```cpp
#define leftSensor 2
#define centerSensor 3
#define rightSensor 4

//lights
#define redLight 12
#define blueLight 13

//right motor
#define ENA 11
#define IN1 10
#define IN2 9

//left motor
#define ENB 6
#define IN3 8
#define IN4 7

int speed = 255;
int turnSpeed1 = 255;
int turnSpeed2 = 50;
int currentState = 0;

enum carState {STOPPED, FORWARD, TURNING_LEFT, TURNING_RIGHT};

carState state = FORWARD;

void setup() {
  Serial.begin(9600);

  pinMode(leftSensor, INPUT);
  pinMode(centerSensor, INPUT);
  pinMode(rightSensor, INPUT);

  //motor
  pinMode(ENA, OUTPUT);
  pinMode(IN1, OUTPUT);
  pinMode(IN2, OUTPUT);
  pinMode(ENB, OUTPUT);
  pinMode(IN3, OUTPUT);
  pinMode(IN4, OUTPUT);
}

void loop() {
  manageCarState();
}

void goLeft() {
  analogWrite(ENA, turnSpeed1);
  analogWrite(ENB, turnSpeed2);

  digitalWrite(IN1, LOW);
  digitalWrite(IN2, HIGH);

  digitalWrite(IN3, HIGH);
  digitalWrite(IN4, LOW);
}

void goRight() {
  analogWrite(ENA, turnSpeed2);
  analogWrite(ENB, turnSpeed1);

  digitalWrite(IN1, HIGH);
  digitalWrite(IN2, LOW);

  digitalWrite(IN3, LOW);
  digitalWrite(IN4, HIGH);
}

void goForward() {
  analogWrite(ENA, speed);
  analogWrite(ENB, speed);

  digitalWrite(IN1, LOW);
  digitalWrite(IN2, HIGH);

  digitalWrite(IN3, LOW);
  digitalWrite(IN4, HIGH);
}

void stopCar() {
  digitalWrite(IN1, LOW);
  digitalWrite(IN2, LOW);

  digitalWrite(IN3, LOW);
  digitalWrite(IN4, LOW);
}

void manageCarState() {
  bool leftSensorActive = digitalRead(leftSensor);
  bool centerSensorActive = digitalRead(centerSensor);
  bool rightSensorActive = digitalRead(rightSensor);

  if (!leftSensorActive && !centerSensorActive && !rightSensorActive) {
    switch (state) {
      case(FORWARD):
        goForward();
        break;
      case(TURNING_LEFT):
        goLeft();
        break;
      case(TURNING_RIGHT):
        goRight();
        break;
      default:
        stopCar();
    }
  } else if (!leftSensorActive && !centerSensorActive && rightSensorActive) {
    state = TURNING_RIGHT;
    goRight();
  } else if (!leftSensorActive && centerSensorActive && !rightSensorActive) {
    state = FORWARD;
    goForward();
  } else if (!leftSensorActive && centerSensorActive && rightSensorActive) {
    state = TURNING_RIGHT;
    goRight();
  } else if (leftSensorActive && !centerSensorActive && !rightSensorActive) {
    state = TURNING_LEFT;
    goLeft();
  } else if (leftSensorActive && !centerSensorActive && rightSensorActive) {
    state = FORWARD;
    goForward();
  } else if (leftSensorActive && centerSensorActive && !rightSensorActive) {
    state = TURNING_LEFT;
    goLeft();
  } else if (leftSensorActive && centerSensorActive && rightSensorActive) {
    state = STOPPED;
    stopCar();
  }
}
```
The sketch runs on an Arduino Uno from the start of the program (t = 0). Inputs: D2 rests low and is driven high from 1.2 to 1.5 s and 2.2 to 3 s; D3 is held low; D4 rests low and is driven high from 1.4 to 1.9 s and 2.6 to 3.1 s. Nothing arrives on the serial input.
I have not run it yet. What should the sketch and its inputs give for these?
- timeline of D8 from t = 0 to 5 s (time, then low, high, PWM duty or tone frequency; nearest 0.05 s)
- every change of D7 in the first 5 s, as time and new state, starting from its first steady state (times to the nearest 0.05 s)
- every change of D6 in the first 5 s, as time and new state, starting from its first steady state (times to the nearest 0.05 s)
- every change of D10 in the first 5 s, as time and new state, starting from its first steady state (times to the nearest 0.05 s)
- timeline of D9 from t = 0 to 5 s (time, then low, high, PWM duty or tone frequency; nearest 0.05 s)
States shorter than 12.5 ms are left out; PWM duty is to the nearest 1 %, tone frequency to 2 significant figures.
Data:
0 s low; 1.2 s high; 1.4 s low; 2.2 s high; 2.6 s low
0 s high; 1.2 s low; 1.4 s high; 2.2 s low; 2.6 s high
0 s high; 1.2 s PWM 20 %; 1.4 s high; 2.2 s PWM 20 %; 2.6 s high
0 s low; 1.5 s high; 2.2 s low; 3 s high
0 s high; 1.5 s low; 2.2 s high; 3 s low
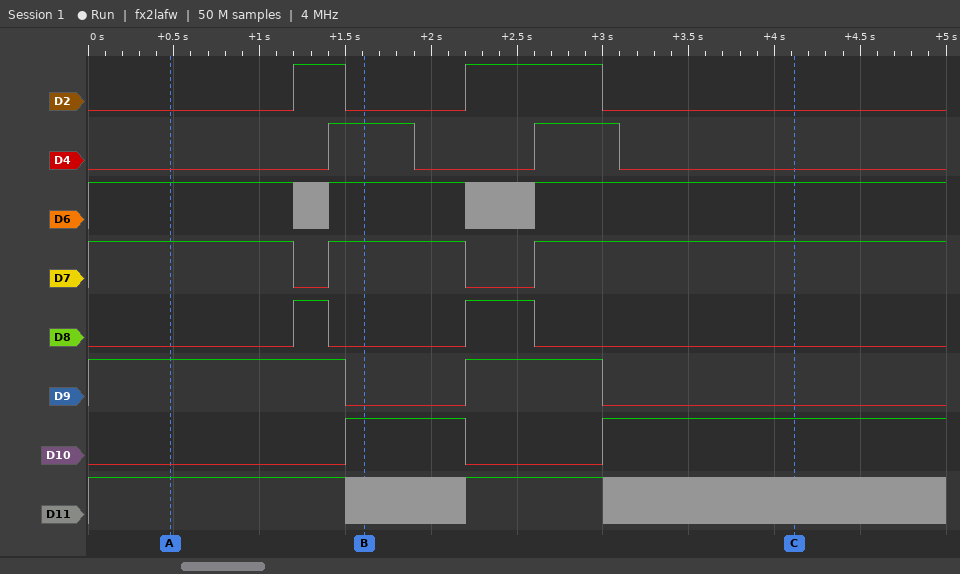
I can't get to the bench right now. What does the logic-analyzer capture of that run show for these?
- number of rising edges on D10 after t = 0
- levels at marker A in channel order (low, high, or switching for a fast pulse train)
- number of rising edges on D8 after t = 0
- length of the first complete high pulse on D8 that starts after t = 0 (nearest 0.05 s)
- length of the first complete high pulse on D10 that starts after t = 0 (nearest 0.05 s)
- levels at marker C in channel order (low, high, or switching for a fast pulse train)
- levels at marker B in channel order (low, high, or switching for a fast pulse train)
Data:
2
D2 low, D4 low, D6 high, D7 high, D8 low, D9 high, D10 low, D11 high
2
0.20 s
0.70 s
D2 low, D4 low, D6 high, D7 high, D8 low, D9 low, D10 high, D11 switching
D2 low, D4 high, D6 high, D7 high, D8 low, D9 low, D10 high, D11 switching
